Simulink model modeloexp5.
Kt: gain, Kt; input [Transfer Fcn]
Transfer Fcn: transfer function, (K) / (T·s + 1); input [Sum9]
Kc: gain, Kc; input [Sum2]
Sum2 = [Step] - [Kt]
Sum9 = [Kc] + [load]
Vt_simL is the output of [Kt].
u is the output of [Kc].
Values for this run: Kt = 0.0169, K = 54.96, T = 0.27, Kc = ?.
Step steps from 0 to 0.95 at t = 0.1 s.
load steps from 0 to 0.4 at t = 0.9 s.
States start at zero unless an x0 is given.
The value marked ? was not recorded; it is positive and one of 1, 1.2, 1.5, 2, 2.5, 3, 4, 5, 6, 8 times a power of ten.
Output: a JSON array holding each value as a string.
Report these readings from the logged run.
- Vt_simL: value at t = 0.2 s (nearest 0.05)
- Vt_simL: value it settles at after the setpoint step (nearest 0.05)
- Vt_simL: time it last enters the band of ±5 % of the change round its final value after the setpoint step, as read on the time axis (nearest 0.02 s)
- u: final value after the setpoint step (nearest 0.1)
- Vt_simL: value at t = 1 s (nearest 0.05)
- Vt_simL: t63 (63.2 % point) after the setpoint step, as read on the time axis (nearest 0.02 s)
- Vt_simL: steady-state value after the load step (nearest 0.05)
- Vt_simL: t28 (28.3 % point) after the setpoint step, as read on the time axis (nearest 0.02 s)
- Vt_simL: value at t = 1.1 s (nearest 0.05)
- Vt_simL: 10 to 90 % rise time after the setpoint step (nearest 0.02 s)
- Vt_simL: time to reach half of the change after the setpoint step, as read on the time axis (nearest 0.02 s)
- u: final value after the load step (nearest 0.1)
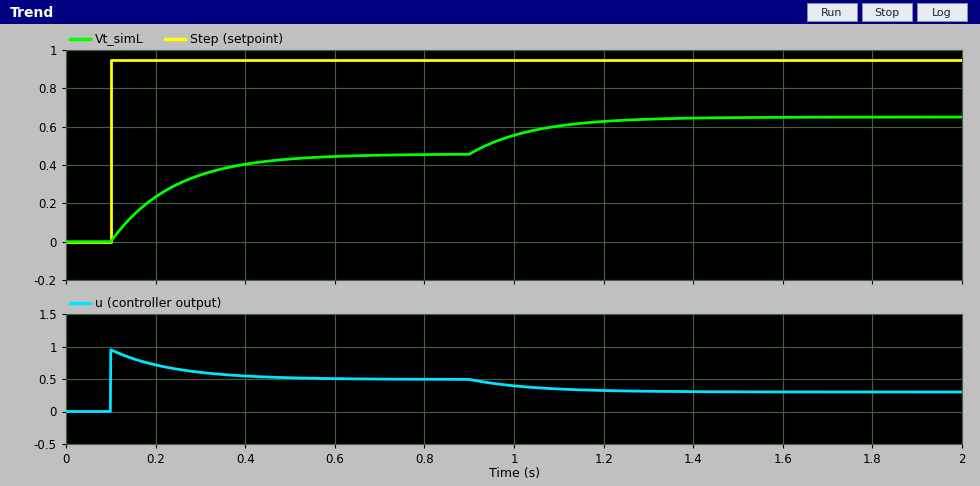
["0.25", "0.45", "0.52 s", "0.5", "0.55", "0.24 s", "0.65", "0.14 s", "0.60", "0.30 s", "0.20 s", "0.3"]
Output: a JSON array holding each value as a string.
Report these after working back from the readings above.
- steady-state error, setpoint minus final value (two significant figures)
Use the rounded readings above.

["0.50"]
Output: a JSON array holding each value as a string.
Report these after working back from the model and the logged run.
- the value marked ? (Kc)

["1"]
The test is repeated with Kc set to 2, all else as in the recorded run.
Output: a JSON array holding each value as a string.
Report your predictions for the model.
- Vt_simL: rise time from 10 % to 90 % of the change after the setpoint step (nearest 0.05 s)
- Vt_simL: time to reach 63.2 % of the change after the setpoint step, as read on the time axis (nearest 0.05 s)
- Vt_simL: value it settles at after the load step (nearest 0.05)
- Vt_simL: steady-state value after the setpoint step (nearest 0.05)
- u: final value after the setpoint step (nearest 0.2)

["0.20 s", "0.20 s", "0.75", "0.60", "0.6"]
